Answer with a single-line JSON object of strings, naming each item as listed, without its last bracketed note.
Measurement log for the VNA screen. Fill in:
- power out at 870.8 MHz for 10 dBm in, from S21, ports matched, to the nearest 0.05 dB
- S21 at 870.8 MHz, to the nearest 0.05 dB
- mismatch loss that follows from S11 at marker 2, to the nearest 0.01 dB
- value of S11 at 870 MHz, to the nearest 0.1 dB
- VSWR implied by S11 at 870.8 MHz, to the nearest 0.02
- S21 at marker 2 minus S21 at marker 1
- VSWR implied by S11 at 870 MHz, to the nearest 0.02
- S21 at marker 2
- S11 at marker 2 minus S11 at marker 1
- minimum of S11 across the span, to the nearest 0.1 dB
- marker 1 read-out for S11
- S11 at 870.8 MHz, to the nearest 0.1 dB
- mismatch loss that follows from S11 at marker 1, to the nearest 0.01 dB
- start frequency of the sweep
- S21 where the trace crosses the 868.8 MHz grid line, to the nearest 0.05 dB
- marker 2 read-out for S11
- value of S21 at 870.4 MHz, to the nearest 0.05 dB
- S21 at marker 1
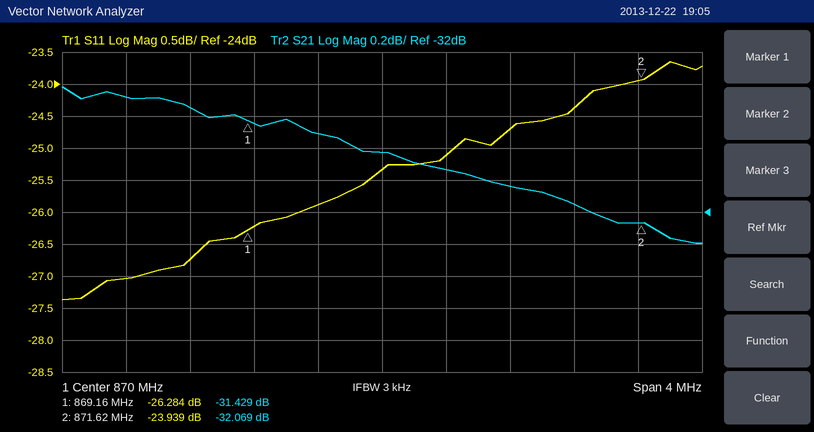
{"power out at 870.8 MHz for 10 dBm in, from S21, ports matched, to the nearest 0.05 dB": "-21.85 dBm", "S21 at 870.8 MHz, to the nearest 0.05 dB": "-31.85 dB", "mismatch loss that follows from S11 at marker 2, to the nearest 0.01 dB": "0.02 dB", "value of S11 at 870 MHz, to the nearest 0.1 dB": "-25.3 dB", "VSWR implied by S11 at 870.8 MHz, to the nearest 0.02": "1.12", "S21 at marker 2 minus S21 at marker 1": "-0.640 dB", "VSWR implied by S11 at 870 MHz, to the nearest 0.02": "1.12", "S21 at marker 2": "-32.069 dB", "S11 at marker 2 minus S11 at marker 1": "2.345 dB", "minimum of S11 across the span, to the nearest 0.1 dB": "-27.4 dB", "marker 1 read-out for S11": "-26.284 dB", "S11 at 870.8 MHz, to the nearest 0.1 dB": "-24.7 dB", "mismatch loss that follows from S11 at marker 1, to the nearest 0.01 dB": "0.01 dB", "start frequency of the sweep": "868 MHz", "S21 where the trace crosses the 868.8 MHz grid line, to the nearest 0.05 dB": "-31.35 dB", "marker 2 read-out for S11": "-23.939 dB", "value of S21 at 870.4 MHz, to the nearest 0.05 dB": "-31.75 dB", "S21 at marker 1": "-31.429 dB"}
